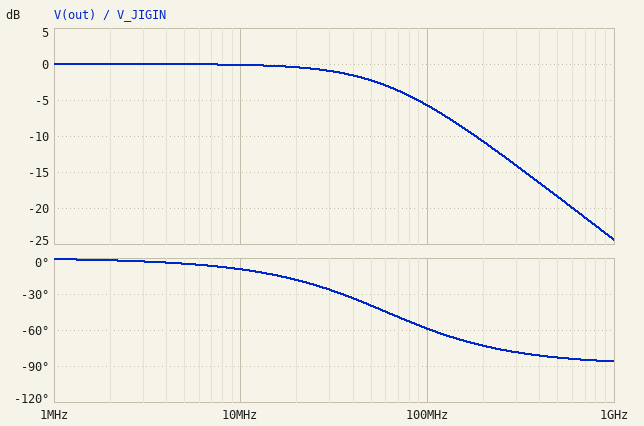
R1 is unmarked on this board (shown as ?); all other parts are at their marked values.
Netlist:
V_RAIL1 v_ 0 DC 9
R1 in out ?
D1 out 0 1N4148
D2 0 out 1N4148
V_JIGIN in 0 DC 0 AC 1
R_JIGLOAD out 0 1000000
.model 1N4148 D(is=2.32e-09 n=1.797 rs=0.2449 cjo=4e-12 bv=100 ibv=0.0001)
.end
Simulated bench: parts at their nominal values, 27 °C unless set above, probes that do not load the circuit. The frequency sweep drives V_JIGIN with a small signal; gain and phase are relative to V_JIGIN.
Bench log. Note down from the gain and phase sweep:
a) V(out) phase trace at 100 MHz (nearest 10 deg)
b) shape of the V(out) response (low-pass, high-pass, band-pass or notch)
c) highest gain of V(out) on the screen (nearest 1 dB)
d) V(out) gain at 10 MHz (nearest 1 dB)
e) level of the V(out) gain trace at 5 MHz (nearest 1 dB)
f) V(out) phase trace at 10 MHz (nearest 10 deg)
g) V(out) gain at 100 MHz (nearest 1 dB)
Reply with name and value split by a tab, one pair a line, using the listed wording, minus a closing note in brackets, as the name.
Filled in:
V(out) phase trace at 100 MHz	-60 deg
shape of the V(out) response	low-pass
highest gain of V(out) on the screen	0 dB
V(out) gain at 10 MHz	0 dB
level of the V(out) gain trace at 5 MHz	0 dB
V(out) phase trace at 10 MHz	-10 deg
V(out) gain at 100 MHz	-6 dB
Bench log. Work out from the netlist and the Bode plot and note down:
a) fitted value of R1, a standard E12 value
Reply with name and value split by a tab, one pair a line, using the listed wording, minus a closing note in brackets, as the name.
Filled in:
fitted value of R1, a standard E12 value	330 Ω
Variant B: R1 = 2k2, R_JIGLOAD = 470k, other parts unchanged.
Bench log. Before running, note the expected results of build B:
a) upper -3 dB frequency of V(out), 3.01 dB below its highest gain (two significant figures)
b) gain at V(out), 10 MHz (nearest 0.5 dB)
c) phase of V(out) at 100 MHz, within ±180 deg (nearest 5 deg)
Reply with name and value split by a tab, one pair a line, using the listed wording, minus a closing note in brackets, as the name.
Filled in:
upper -3 dB frequency of V(out), 3.01 dB below its highest gain	9.1 MHz
gain at V(out), 10 MHz	-3.5 dB
phase of V(out) at 100 MHz, within ±180 deg	-85 deg
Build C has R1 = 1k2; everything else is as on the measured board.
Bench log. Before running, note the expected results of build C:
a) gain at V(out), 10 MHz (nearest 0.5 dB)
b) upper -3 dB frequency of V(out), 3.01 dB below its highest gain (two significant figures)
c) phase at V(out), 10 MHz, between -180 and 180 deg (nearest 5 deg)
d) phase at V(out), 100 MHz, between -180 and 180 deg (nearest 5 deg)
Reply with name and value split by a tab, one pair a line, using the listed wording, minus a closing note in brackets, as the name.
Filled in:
gain at V(out), 10 MHz	-1.5 dB
upper -3 dB frequency of V(out), 3.01 dB below its highest gain	17 MHz
phase at V(out), 10 MHz, between -180 and 180 deg	-30 deg
phase at V(out), 100 MHz, between -180 and 180 deg	-80 deg
